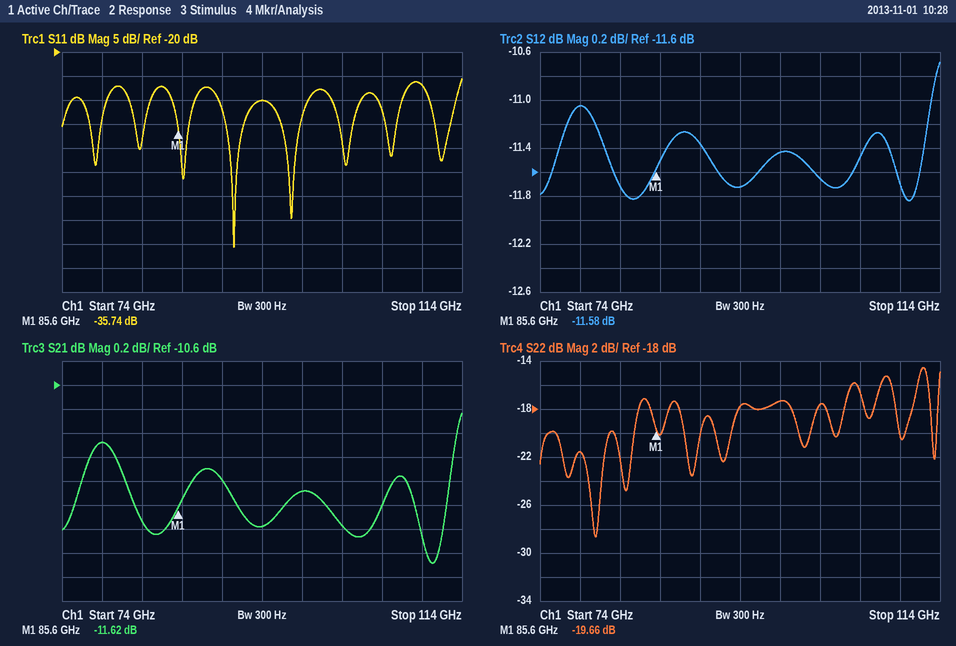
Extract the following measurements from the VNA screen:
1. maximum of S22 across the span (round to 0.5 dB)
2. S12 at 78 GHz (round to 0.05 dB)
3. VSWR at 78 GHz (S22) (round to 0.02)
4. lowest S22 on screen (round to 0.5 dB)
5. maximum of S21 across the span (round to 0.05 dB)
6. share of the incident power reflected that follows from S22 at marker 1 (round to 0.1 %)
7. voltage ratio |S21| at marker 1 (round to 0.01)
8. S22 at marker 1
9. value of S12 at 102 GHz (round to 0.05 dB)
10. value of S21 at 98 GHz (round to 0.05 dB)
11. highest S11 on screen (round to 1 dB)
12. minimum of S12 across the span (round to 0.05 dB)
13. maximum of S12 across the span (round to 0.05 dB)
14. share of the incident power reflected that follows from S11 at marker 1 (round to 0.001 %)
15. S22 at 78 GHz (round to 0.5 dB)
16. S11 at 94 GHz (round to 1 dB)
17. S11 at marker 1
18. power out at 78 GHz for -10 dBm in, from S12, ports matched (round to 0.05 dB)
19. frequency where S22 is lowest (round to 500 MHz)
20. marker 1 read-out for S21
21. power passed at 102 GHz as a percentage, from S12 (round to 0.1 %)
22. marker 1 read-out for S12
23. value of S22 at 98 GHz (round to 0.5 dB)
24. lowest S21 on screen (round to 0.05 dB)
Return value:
-14.5 dB
-11.05 dB
1.18
-28.5 dB
-10.85 dB
1.1 %
0.26
-19.66 dB
-11.65 dB
-11.50 dB
-26 dB
-11.85 dB
-10.70 dB
0.027 %
-21.5 dB
-30 dB
-35.74 dB
-21.05 dBm
79.5 GHz
-11.62 dB
6.8 %
-11.58 dB
-17.5 dB
-12.10 dB
